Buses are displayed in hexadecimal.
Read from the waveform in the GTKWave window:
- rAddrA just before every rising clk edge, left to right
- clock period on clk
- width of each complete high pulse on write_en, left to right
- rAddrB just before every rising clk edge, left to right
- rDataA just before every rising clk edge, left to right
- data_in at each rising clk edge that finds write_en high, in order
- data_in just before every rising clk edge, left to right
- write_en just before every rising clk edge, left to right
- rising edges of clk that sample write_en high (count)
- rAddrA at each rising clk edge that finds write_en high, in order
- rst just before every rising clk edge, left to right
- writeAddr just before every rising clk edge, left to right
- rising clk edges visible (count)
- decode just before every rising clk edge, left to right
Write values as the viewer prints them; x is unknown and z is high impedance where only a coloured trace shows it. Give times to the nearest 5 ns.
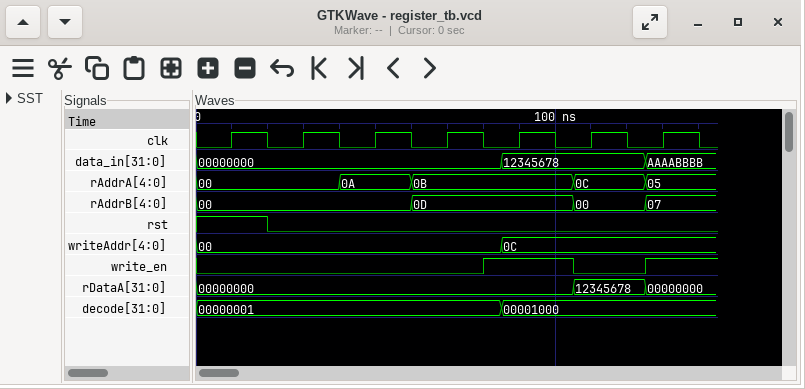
00, 00, 0A, 0B, 0B, 0C, 05
20 ns
25 ns
00, 00, 00, 0D, 0D, 00, 07
00000000, 00000000, 00000000, 00000000, 00000000, 12345678, 00000000
12345678, AAAABBBB
00000000, 00000000, 00000000, 00000000, 12345678, 12345678, AAAABBBB
0 0 0 0 1 0 1
2
0B, 05
1 0 0 0 0 0 0
00, 00, 00, 00, 0C, 0C, 0C
7
00000001, 00000001, 00000001, 00000001, 00001000, 00001000, 00001000
